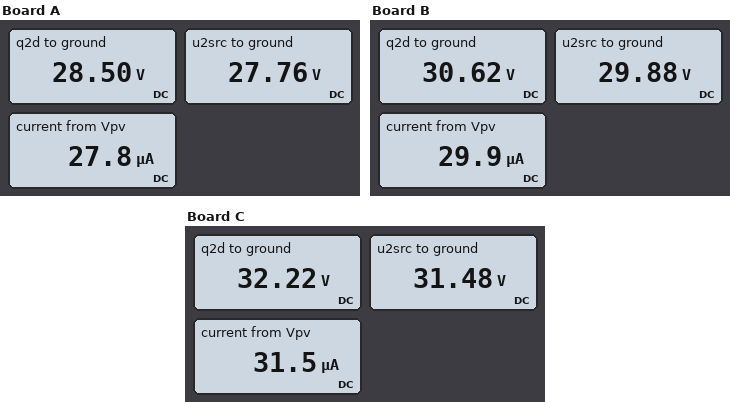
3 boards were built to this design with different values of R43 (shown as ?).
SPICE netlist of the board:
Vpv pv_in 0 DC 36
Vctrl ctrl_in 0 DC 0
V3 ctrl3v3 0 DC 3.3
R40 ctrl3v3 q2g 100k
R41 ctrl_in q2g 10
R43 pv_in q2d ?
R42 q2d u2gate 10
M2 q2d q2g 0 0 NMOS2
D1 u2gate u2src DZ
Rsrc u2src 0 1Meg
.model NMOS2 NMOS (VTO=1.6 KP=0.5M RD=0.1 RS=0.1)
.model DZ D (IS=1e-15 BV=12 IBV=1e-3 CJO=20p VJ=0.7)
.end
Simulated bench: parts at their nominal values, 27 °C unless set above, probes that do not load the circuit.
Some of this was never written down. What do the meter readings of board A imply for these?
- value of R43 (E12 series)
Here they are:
270 kΩ
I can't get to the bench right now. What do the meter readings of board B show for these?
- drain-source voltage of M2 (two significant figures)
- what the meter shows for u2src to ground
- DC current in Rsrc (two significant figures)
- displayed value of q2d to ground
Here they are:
31 V
29.88 V
30 µA
30.62 V
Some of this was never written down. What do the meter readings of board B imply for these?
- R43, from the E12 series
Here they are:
180 kΩ
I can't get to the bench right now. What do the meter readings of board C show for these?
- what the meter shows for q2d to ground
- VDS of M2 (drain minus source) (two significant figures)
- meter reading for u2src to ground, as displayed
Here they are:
32.22 V
32 V
31.48 V
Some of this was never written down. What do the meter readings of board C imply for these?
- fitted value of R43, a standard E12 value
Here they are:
120 kΩ
